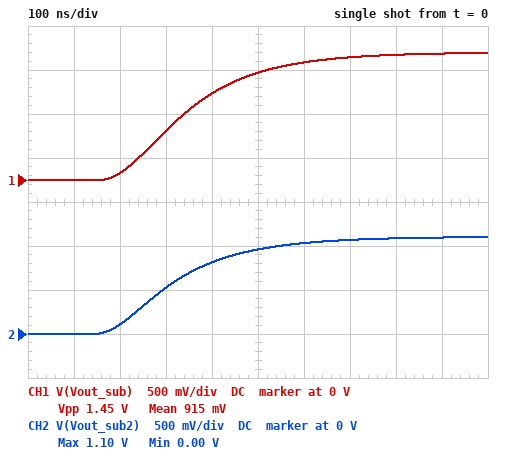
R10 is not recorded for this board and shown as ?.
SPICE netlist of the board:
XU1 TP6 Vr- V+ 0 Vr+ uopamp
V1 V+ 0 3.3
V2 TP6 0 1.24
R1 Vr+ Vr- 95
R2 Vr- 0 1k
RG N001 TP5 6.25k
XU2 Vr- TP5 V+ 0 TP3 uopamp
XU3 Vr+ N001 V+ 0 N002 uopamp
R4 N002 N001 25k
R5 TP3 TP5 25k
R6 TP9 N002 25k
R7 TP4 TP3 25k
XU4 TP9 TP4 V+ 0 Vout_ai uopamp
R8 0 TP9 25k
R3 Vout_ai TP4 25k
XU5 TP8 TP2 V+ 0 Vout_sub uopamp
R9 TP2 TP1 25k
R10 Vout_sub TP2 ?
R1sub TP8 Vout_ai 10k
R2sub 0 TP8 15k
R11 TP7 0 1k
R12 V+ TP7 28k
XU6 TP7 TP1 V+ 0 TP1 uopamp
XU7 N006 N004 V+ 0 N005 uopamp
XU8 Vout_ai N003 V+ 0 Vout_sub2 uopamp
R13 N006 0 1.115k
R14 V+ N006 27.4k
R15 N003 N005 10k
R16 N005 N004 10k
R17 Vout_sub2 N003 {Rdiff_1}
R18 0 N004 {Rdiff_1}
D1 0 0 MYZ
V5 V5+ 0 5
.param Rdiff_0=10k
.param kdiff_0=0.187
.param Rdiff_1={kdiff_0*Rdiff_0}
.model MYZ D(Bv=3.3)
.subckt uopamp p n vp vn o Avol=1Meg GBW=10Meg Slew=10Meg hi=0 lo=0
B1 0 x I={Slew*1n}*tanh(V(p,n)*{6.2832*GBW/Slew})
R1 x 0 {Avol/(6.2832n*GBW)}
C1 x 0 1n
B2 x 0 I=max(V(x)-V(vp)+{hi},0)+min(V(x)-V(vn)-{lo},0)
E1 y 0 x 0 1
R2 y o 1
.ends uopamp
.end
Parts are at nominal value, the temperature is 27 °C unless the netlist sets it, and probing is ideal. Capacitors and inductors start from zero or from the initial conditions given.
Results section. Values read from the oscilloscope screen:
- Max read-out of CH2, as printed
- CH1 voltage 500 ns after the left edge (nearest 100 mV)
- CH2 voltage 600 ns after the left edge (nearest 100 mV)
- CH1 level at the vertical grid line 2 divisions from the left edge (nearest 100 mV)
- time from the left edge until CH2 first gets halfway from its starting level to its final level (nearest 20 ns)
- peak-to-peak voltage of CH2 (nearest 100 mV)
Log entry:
1.10 V
1.2 V
1.0 V
100 mV
300 ns
1.1 V
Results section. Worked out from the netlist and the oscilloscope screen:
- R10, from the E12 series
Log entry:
39 kΩ
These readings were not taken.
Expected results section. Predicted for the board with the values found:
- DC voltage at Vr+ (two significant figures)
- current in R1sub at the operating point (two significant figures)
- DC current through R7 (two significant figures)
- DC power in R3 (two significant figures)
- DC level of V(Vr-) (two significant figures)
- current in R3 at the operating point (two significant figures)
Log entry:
1.4 V
42 µA
5.8 µA
850 nW
1.2 V
5.8 µA
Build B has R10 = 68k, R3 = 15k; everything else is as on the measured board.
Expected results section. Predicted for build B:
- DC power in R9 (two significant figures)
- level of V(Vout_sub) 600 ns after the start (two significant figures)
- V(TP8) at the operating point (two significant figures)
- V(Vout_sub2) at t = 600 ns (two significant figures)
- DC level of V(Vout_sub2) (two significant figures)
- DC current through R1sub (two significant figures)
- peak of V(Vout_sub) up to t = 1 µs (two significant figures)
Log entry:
9.5 µW
1.8 V
600 mV
990 mV
1.0 V
40 µA
1.9 V
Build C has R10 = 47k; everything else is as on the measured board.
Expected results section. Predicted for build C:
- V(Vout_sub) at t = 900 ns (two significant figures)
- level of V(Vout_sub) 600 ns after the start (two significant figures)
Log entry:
1.6 V
1.5 V
